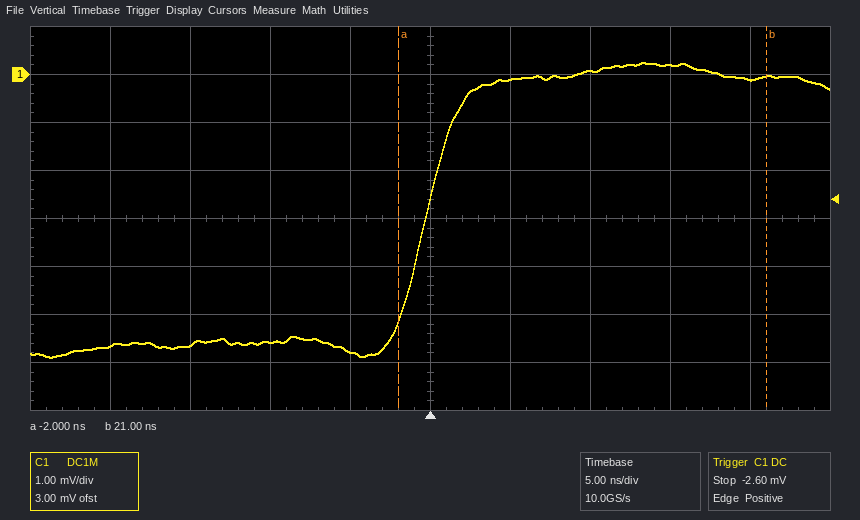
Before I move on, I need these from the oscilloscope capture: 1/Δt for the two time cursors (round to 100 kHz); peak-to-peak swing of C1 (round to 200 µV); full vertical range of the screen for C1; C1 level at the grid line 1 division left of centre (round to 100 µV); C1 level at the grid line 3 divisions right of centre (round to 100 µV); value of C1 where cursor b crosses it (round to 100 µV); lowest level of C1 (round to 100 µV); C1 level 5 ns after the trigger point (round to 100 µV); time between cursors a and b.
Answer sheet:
43.5 MHz
6.2 mV
8 mV
-5.8 mV
200 µV
0.0 mV
-5.9 mV
-100 µV
23.0 ns
